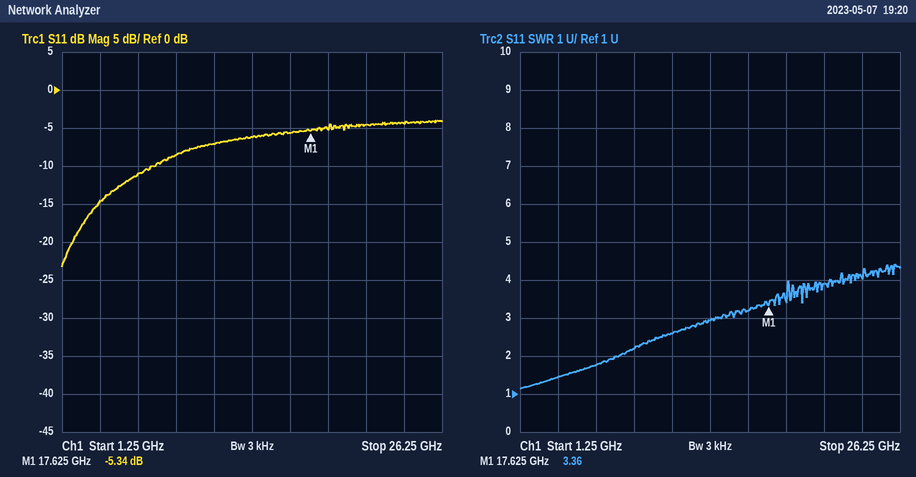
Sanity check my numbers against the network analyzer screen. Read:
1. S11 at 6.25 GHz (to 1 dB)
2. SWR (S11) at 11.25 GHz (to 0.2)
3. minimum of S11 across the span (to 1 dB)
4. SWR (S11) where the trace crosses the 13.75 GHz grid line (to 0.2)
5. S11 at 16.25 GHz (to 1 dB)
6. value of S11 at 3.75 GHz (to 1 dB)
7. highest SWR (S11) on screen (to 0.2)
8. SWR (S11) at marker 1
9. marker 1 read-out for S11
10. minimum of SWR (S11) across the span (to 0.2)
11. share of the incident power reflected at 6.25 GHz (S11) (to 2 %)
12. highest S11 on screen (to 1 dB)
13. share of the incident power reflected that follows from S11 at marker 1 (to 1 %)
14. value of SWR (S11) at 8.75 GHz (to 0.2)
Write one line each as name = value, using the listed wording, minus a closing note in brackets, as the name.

S11 at 6.25 GHz = -11 dB
SWR (S11) at 11.25 GHz = 2.6
minimum of S11 across the span = -23 dB
SWR (S11) where the trace crosses the 13.75 GHz grid line = 3.0
S11 at 16.25 GHz = -6 dB
value of S11 at 3.75 GHz = -15 dB
highest SWR (S11) on screen = 4.4
SWR (S11) at marker 1 = 3.36
marker 1 read-out for S11 = -5.34 dB
minimum of SWR (S11) across the span = 1.2
share of the incident power reflected at 6.25 GHz (S11) = 8 %
highest S11 on screen = -4 dB
share of the incident power reflected that follows from S11 at marker 1 = 29 %
value of SWR (S11) at 8.75 GHz = 2.2
